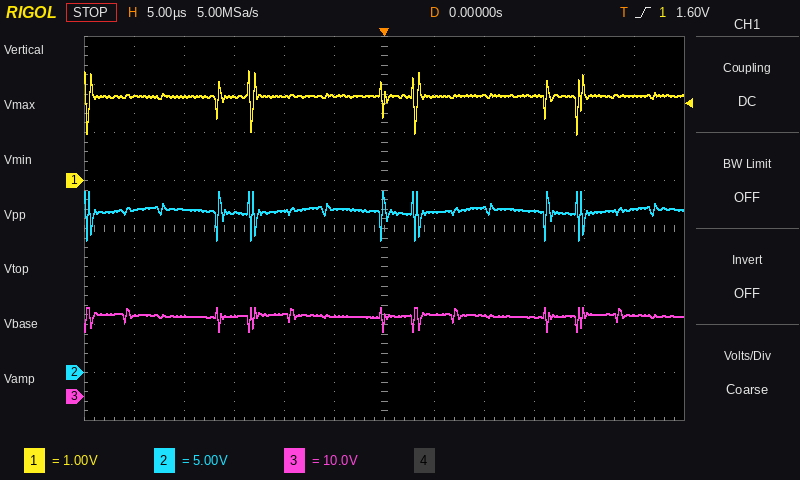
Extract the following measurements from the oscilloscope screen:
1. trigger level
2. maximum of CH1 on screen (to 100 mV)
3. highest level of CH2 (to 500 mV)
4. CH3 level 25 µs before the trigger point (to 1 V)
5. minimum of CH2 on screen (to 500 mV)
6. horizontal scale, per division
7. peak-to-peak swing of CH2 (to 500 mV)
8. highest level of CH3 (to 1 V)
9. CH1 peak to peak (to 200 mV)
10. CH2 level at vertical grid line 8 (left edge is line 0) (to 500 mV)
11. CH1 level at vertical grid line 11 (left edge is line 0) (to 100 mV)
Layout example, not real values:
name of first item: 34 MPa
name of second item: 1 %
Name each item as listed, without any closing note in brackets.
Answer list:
trigger level: 1.60 V
maximum of CH1 on screen: 2.3 V
highest level of CH2: 19.0 V
CH3 level 25 µs before the trigger point: 17 V
minimum of CH2 on screen: 14.0 V
horizontal scale, per division: 5 µs
peak-to-peak swing of CH2: 5.0 V
highest level of CH3: 19 V
CH1 peak to peak: 1.4 V
CH2 level at vertical grid line 8 (left edge is line 0): 17.0 V
CH1 level at vertical grid line 11 (left edge is line 0): 1.8 V
